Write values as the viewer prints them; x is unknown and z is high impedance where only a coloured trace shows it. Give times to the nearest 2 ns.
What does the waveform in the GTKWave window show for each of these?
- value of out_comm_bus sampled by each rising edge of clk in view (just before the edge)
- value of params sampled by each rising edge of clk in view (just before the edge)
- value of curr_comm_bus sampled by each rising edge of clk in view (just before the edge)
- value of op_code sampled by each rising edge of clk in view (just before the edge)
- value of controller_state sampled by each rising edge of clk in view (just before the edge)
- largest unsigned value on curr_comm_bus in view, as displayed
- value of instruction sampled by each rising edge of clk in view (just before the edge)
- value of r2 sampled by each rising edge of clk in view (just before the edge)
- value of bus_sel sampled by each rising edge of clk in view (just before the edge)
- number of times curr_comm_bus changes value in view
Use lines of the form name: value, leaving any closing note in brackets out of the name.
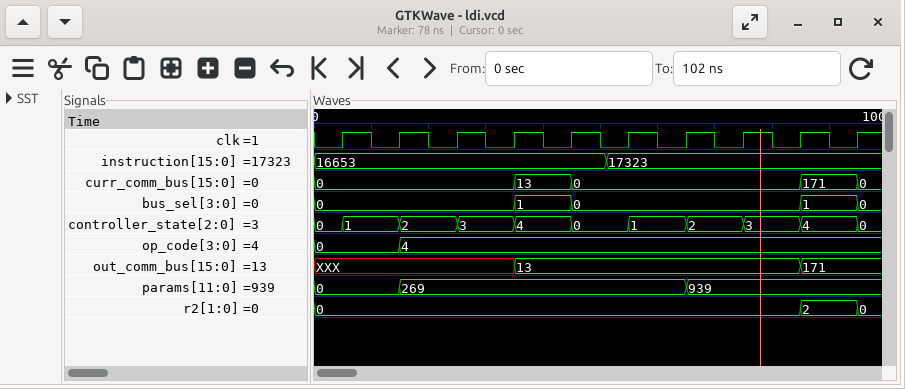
value of out_comm_bus sampled by each rising edge of clk in view: XXX, XXX, XXX, XXX, 13, 13, 13, 13, 13, 171
value of params sampled by each rising edge of clk in view: 0, 0, 269, 269, 269, 269, 269, 939, 939, 939
value of curr_comm_bus sampled by each rising edge of clk in view: 0, 0, 0, 0, 13, 0, 0, 0, 0, 171
value of op_code sampled by each rising edge of clk in view: 0, 0, 4, 4, 4, 4, 4, 4, 4, 4
value of controller_state sampled by each rising edge of clk in view: 0, 1, 2, 3, 4, 0, 1, 2, 3, 4
largest unsigned value on curr_comm_bus in view, as displayed: 171
value of instruction sampled by each rising edge of clk in view: 16653, 16653, 16653, 16653, 16653, 17323, 17323, 17323, 17323, 17323
value of r2 sampled by each rising edge of clk in view: 0, 0, 0, 0, 0, 0, 0, 0, 0, 2
value of bus_sel sampled by each rising edge of clk in view: 0, 0, 0, 0, 1, 0, 0, 0, 0, 1
number of times curr_comm_bus changes value in view: 4
